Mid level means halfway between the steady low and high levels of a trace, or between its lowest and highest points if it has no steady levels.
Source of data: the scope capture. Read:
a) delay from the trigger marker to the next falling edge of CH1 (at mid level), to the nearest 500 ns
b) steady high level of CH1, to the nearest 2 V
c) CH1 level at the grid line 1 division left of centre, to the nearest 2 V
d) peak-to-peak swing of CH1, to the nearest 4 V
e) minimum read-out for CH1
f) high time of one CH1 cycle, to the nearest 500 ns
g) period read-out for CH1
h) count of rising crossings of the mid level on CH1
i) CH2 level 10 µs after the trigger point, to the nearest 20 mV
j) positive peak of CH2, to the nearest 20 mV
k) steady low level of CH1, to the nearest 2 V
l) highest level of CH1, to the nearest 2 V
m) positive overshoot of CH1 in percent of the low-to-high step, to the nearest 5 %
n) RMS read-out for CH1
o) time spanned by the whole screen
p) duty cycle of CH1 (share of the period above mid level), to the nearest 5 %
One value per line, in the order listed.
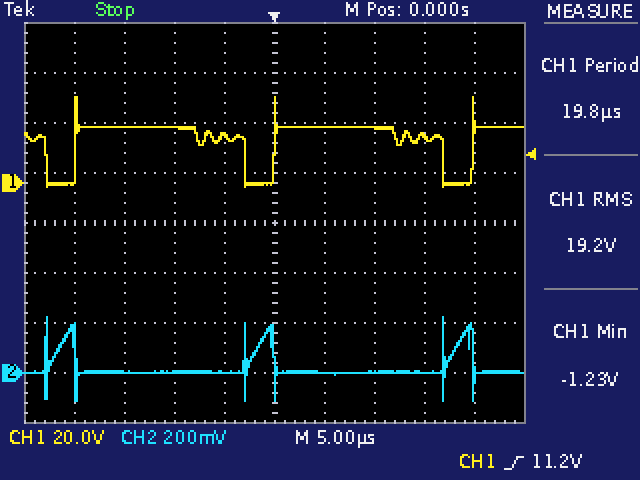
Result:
17.0 µs
22 V
18 V
36 V
-1.23 V
17.0 µs
19.8 µs
3
0 mV
220 mV
0 V
34 V
55 %
19.2 V
50 µs
85 %
